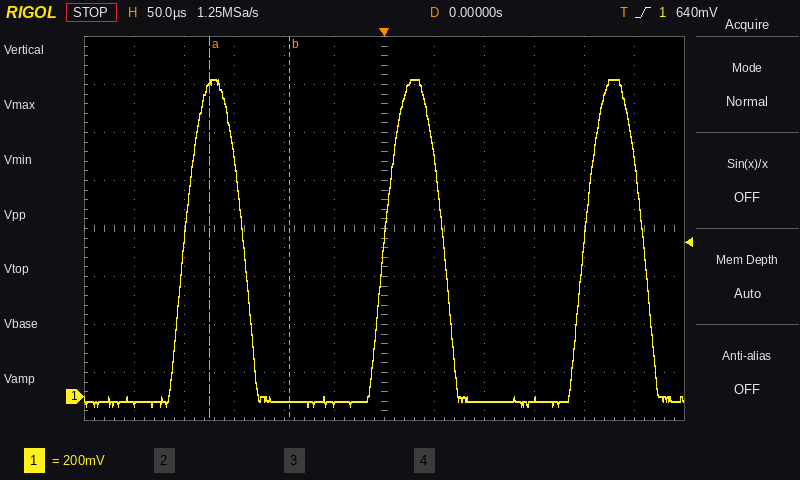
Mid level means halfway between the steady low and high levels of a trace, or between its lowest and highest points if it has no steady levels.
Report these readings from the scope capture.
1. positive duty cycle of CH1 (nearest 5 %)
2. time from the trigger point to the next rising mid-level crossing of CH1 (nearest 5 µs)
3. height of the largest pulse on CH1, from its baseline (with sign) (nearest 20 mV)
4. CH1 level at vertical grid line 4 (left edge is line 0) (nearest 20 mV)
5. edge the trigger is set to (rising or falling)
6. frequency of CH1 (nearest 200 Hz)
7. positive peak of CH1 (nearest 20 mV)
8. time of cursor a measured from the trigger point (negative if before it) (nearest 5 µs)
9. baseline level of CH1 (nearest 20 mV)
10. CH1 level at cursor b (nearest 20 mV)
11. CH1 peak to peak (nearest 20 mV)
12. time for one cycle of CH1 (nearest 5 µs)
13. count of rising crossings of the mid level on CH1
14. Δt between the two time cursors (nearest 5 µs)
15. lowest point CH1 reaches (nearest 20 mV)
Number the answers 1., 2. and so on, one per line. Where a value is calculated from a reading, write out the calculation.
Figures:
1. 30 %
2. 200 µs
3. 1.32 V − (-20 mV) = +1.34 V
4. -20 mV
5. rising
6. 1 / 200 µs ≈ 5.0 kHz
7. 1.32 V
8. -175 µs
9. -20 mV
10. -20 mV
11. 1.32 V − (-40 mV) = 1.36 V
12. 200 µs
13. 3
14. 80 µs
15. -40 mV
